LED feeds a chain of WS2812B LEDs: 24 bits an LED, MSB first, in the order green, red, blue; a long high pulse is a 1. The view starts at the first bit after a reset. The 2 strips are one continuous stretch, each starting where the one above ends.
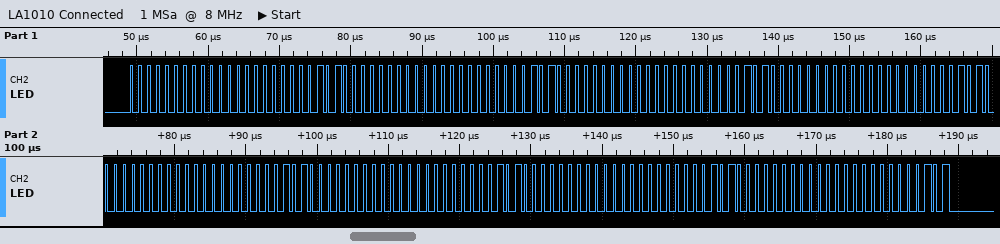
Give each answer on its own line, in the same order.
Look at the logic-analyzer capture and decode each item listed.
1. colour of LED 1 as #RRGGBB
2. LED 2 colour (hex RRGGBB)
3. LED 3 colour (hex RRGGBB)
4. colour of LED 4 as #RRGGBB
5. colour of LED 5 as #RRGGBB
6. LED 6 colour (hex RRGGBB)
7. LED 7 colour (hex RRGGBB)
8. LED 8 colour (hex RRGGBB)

#000005
#000005
#000005
#000005
#000005
#000005
#000005
#000005
